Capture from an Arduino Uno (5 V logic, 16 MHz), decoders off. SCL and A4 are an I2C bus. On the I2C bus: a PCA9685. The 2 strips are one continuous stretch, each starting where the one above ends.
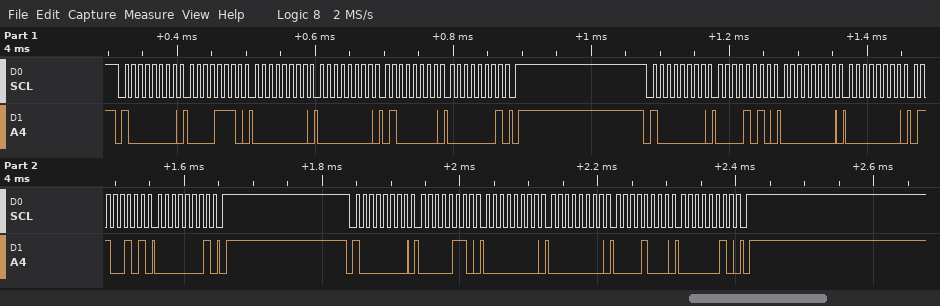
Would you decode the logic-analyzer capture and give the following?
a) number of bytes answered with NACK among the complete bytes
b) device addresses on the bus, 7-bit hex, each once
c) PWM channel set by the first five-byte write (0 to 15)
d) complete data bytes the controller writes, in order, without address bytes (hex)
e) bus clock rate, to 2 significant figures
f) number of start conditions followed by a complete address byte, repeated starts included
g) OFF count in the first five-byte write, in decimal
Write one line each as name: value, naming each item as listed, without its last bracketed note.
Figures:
number of bytes answered with NACK among the complete bytes: 0
device addresses on the bus, 7-bit hex, each once: 0x40
PWM channel set by the first five-byte write: 2
complete data bytes the controller writes, in order, without address bytes: 0E 00 00 40 01 0A 00 00 65 01 06 00 00 08 02
bus clock rate, to 2 significant figures: 100 kHz
number of start conditions followed by a complete address byte, repeated starts included: 3
OFF count in the first five-byte write, in decimal: 320
